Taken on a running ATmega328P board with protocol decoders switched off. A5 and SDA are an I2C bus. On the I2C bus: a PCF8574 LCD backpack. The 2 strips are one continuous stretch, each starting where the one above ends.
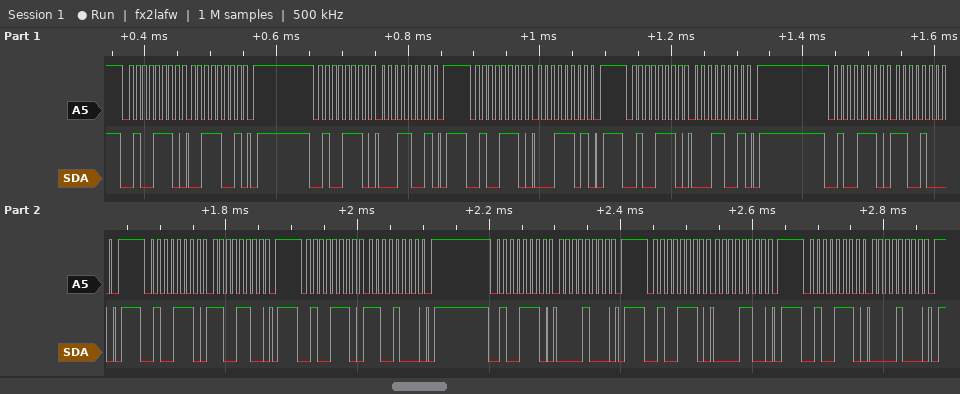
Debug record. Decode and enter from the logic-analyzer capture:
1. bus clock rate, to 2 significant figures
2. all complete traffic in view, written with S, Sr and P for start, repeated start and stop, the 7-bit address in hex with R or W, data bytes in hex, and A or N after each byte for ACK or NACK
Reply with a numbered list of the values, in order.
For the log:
1. 100 kHz
2. S 27W A 39 A P S 27W A 19 A P S 27W A 1D A P S 27W A 19 A P S 27W A C8 A P S 27W A CC A P S 27W A C8 A P S 27W A 08 A P S 27W A 0C A P S 27W A 08 A P
